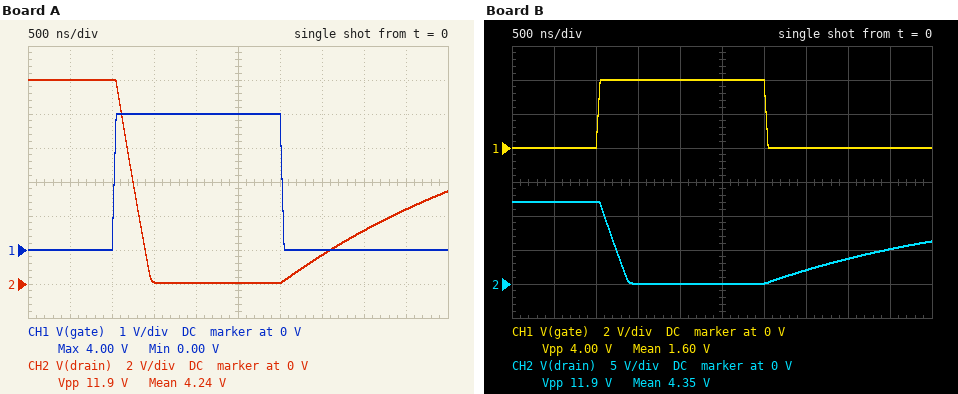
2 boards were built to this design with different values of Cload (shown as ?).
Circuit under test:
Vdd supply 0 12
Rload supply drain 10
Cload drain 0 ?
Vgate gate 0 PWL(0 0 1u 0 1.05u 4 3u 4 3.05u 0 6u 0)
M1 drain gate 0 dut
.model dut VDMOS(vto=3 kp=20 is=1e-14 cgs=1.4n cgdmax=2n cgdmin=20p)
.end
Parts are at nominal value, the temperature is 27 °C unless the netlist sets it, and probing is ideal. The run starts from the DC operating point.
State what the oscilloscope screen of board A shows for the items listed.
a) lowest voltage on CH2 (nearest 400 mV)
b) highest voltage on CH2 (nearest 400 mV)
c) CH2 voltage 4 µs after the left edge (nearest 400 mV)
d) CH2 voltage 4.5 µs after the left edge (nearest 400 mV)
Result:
0 V
12.0 V
3.2 V
4.4 V
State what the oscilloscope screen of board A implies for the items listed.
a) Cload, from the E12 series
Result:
330 nF
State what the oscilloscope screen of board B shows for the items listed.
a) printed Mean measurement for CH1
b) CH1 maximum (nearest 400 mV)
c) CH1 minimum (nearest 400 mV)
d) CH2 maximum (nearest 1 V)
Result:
1.60 V
4.0 V
0 V
12 V
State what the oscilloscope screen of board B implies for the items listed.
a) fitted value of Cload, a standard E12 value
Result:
270 nF
